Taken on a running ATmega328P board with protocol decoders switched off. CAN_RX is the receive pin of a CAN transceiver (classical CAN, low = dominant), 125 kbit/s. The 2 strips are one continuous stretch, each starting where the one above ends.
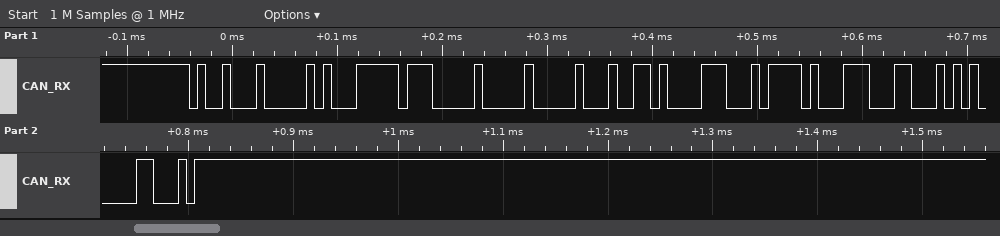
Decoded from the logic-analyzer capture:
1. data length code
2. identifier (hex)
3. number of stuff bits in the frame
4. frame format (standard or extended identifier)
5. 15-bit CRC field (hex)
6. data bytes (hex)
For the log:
8
0x488
6
standard
0x2A08
FF 00 00 26 87 17 A3 8C
